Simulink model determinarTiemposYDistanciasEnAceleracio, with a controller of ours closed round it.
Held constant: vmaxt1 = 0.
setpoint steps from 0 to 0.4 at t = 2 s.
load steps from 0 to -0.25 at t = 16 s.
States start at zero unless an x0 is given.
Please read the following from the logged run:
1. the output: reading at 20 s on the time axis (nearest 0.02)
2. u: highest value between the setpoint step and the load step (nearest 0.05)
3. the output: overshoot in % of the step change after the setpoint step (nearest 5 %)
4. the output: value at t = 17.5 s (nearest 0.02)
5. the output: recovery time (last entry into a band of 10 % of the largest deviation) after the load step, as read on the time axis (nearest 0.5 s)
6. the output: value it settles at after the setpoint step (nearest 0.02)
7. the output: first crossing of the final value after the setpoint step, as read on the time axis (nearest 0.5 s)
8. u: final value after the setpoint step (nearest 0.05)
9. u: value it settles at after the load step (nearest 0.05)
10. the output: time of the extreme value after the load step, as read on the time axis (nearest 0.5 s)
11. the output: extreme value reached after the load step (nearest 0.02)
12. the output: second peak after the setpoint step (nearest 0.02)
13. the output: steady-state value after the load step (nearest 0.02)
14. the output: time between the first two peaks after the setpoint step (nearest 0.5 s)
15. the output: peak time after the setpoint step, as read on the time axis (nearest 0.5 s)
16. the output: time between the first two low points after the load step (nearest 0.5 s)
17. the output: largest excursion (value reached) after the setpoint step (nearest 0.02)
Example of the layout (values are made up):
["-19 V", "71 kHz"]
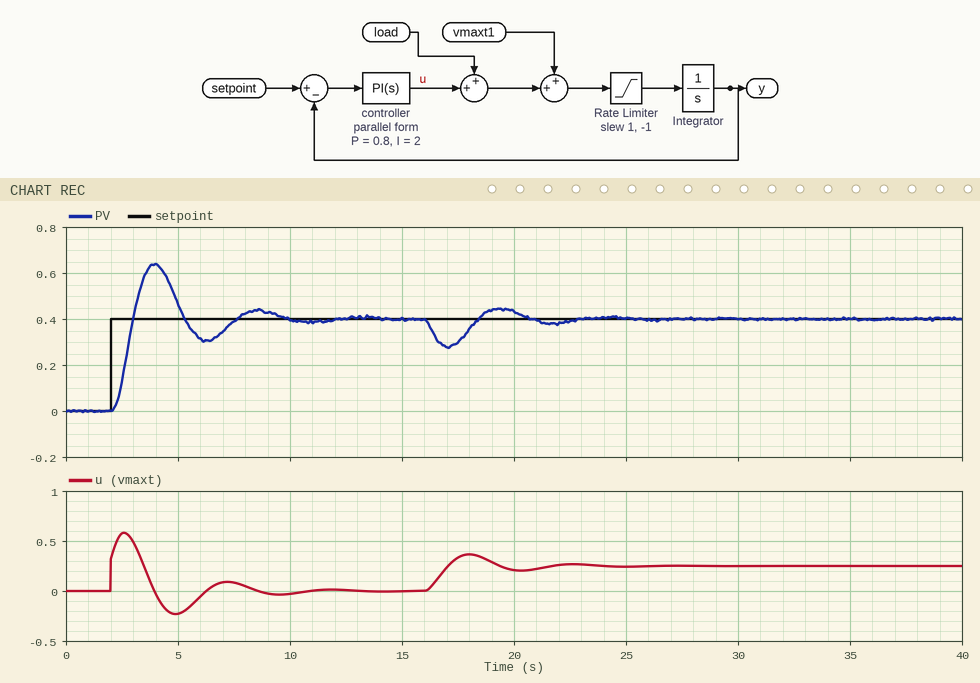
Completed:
["0.44", "0.60", "60 %", "0.30", "22.5 s", "0.40", "3.0 s", "0.00", "0.25", "17.0 s", "0.28", "0.44", "0.40", "4.5 s", "4.0 s", "4.5 s", "0.64"]
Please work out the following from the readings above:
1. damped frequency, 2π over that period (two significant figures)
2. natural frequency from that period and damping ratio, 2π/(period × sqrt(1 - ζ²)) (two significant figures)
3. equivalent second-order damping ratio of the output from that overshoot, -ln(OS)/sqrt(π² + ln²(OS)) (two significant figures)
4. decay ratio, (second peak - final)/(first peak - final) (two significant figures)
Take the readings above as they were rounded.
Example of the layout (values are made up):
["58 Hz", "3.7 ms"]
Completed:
["1.4 rad/s", "1.4 rad/s", "0.16", "0.17"]
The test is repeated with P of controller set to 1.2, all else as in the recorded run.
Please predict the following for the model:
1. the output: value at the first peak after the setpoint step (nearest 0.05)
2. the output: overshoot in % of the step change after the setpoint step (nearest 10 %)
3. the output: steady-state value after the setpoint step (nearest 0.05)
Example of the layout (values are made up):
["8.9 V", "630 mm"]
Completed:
["0.60", "50 %", "0.40"]
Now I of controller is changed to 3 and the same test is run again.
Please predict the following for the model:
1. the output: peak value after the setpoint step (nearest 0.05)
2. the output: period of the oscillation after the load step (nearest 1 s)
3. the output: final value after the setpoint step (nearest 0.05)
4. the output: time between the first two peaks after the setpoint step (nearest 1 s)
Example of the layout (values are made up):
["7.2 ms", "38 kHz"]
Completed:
["0.70", "4 s", "0.40", "4 s"]
